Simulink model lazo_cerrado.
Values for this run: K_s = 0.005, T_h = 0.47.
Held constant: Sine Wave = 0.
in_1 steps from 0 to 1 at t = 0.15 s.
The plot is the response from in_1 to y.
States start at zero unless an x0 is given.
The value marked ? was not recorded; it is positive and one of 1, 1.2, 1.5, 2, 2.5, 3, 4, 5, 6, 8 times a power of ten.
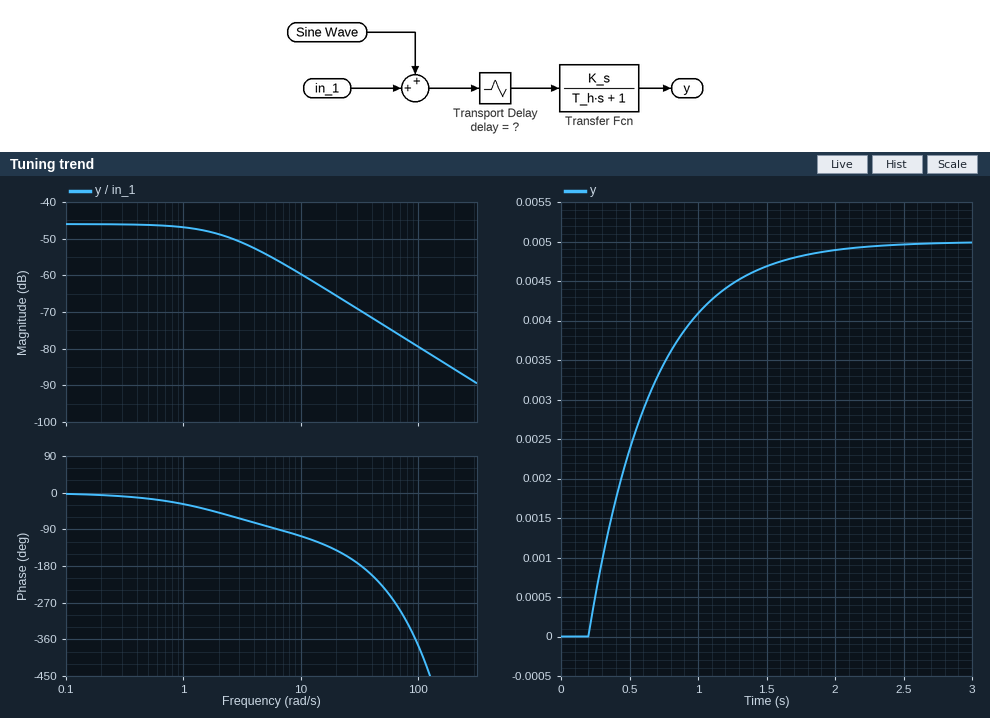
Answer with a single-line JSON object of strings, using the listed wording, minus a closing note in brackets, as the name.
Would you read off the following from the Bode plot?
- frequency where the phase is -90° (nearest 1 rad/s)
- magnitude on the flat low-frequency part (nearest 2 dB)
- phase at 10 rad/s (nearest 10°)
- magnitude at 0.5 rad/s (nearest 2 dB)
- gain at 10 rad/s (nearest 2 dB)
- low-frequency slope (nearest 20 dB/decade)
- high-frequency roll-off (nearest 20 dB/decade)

{"frequency where the phase is -90°": "6 rad/s", "magnitude on the flat low-frequency part": "-46 dB", "phase at 10 rad/s": "-110°", "magnitude at 0.5 rad/s": "-46 dB", "gain at 10 rad/s": "-60 dB", "low-frequency slope": "0 dB/decade", "high-frequency roll-off": "-20 dB/decade"}
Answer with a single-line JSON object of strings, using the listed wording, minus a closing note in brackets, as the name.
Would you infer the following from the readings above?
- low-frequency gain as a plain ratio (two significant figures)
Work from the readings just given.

{"low-frequency gain as a plain ratio": "0.0050"}
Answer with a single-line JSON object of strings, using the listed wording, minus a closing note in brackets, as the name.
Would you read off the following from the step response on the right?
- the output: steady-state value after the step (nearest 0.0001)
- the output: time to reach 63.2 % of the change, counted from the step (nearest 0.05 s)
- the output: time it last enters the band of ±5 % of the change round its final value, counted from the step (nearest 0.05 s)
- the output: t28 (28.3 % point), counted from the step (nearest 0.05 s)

{"the output: steady-state value after the step": "0.0050", "the output: time to reach 63.2 % of the change, counted from the step": "0.50 s", "the output: time it last enters the band of ±5 % of the change round its final value, counted from the step": "1.45 s", "the output: t28 (28.3 % point), counted from the step": "0.20 s"}
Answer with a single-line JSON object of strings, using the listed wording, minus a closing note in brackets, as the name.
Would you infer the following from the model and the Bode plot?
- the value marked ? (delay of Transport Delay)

{"the value marked ?": "0.05"}
